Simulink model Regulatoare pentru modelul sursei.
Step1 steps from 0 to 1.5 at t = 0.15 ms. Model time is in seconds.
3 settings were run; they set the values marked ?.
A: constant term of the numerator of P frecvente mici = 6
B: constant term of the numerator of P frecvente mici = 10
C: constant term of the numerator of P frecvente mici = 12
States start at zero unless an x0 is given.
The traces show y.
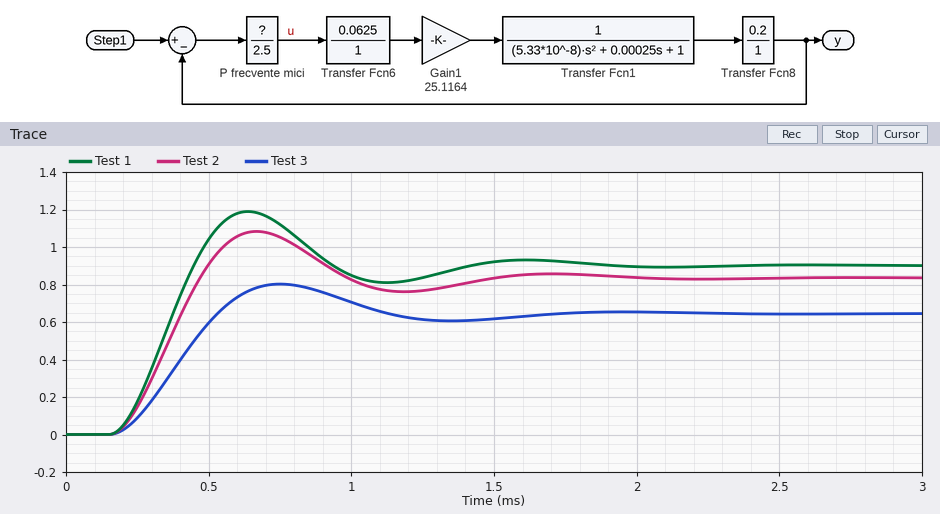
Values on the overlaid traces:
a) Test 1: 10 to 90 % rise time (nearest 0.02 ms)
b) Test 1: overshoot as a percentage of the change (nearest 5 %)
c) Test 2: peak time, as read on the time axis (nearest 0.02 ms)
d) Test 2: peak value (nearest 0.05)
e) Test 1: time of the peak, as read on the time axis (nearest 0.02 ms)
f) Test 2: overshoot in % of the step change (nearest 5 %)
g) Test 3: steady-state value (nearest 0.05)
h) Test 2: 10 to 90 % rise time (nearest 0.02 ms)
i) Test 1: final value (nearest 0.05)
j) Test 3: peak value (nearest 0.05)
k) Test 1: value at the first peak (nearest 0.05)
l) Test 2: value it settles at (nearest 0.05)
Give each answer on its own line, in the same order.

0.20 ms
30 %
0.66 ms
1.10
0.64 ms
30 %
0.65
0.22 ms
0.90
0.80
1.20
0.85
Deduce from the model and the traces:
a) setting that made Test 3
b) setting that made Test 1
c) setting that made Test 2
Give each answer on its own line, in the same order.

A
C
B
